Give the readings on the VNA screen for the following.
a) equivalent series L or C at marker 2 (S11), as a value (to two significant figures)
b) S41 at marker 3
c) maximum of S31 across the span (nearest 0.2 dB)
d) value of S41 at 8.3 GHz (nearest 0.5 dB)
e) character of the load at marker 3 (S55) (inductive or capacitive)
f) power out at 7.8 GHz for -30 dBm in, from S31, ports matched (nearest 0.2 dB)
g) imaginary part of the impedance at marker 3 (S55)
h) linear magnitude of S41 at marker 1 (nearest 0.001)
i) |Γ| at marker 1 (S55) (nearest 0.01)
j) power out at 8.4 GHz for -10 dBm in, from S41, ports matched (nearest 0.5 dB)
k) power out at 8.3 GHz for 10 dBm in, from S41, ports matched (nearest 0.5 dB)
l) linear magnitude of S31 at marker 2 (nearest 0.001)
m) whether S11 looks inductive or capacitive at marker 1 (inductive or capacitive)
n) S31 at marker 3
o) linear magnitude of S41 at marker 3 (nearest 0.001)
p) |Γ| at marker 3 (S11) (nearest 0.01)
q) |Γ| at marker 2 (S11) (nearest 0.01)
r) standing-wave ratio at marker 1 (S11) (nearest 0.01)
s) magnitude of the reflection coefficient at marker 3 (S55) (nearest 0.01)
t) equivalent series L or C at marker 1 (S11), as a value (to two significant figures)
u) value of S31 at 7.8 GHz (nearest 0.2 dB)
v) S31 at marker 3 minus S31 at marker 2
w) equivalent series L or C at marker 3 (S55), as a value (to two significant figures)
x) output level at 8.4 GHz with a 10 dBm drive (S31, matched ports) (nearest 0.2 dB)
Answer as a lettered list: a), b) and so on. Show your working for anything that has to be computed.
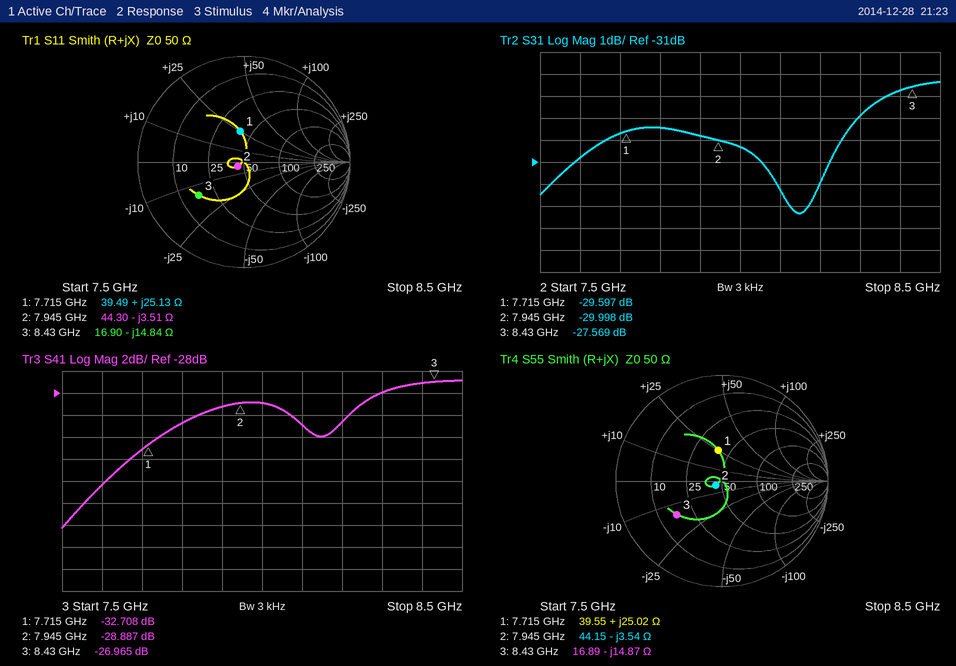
a) C = 1/(2π × 7.945 GHz × 3.51 Ω) ≈ 5.7 pF
b) -26.965 dB
c) -27.4 dB
d) -28.0 dB
e) capacitive
f) -30 dBm + (-29.4 dB) = -59.4 dBm
g) -14.87 Ω
h) 10^(-32.708/20) ≈ 0.023
i) 0.29
j) -10 dBm + (-27.0 dB) = -37.0 dBm
k) 10 dBm + (-28.0 dB) = -18.0 dBm
l) 10^(-29.998/20) ≈ 0.032
m) inductive
n) -27.569 dB
o) 10^(-26.965/20) ≈ 0.045
p) 0.53
q) 0.07
r) 1.83
s) 0.53
t) L = 25.13 Ω/(2π × 7.715 GHz) ≈ 518 pH, so 520 pH to two significant figures
u) -29.4 dB
v) -27.569 − (-29.998) = 2.429 dB
w) C = 1/(2π × 8.43 GHz × 14.87 Ω) ≈ 1.3 pF
x) 10 dBm + (-27.8 dB) = -17.8 dBm
